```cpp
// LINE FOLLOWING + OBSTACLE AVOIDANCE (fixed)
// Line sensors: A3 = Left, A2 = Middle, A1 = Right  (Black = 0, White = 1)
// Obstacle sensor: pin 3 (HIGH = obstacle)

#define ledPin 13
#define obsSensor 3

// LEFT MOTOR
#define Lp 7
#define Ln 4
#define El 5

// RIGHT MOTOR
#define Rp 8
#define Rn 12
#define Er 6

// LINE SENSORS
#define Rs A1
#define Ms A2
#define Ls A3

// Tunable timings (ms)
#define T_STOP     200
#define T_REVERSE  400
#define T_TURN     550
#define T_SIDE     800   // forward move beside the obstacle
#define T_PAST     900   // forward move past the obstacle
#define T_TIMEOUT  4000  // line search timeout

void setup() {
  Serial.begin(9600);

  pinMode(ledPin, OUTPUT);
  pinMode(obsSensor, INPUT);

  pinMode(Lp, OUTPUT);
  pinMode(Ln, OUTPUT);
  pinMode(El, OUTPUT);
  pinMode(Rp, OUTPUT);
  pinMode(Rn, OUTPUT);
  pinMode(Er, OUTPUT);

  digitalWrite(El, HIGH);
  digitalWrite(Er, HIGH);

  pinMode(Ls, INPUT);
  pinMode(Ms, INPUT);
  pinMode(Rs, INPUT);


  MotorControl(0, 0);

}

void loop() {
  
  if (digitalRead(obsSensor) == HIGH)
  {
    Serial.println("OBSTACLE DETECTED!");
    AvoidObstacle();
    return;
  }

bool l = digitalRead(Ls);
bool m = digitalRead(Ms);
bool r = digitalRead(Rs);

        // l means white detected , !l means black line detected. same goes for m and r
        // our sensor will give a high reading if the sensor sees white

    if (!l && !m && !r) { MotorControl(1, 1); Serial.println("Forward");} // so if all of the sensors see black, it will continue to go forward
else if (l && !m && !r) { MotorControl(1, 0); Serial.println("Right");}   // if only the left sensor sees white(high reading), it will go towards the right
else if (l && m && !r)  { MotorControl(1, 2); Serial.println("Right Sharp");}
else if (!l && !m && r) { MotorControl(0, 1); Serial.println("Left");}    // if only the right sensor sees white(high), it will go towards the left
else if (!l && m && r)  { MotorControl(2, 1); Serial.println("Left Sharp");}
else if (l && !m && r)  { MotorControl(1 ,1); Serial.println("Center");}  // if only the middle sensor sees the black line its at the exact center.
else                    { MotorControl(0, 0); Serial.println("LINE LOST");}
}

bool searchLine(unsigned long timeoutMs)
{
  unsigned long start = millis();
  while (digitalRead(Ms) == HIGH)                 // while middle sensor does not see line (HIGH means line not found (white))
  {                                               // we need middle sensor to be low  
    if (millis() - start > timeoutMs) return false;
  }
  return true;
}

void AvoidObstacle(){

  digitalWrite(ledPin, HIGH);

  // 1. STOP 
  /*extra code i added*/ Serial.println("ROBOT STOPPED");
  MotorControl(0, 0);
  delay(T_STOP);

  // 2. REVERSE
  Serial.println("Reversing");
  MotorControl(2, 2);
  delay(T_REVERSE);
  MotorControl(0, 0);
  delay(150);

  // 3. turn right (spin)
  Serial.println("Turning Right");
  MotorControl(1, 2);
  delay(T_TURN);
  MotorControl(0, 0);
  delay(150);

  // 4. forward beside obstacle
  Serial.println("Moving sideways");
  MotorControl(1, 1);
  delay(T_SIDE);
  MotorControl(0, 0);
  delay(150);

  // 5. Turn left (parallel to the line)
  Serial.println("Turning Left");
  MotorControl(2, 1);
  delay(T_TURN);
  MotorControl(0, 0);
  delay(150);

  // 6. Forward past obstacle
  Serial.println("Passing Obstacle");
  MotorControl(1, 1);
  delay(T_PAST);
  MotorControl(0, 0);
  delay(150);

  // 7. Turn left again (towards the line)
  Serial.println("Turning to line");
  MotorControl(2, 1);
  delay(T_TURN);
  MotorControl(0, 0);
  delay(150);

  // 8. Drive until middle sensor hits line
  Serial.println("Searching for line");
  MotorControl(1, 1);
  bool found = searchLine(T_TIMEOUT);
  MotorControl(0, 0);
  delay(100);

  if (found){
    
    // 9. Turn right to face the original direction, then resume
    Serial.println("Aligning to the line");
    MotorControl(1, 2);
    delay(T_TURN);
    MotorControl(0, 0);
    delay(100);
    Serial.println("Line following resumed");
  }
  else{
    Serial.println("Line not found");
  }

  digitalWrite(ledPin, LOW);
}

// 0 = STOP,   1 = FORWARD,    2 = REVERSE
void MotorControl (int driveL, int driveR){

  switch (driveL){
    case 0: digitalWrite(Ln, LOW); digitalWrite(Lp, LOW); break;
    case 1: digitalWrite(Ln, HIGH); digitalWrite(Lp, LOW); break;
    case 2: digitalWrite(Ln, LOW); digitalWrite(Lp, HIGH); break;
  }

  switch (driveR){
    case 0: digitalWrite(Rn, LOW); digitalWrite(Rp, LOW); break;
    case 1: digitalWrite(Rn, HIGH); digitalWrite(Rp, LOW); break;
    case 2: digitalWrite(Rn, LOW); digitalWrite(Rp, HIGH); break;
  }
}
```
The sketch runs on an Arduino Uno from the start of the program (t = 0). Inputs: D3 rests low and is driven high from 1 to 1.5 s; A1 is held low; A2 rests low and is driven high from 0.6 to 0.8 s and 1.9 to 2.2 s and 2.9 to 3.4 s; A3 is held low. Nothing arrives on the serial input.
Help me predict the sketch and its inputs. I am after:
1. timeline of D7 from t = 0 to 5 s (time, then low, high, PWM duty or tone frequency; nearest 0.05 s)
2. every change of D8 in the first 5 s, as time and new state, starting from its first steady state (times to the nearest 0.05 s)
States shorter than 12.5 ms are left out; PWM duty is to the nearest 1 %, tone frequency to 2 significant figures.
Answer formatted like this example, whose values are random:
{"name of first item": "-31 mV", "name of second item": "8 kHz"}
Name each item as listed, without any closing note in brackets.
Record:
{"timeline of D7 from t = 0 to 5 s": "0 s low; 1.25 s high; 1.65 s low; 3.45 s high; 4 s low", "every change of D8 in the first 5 s, as time and new state, starting from its first steady state": "0 s low; 1.25 s high; 1.65 s low; 1.8 s high; 2.35 s low"}
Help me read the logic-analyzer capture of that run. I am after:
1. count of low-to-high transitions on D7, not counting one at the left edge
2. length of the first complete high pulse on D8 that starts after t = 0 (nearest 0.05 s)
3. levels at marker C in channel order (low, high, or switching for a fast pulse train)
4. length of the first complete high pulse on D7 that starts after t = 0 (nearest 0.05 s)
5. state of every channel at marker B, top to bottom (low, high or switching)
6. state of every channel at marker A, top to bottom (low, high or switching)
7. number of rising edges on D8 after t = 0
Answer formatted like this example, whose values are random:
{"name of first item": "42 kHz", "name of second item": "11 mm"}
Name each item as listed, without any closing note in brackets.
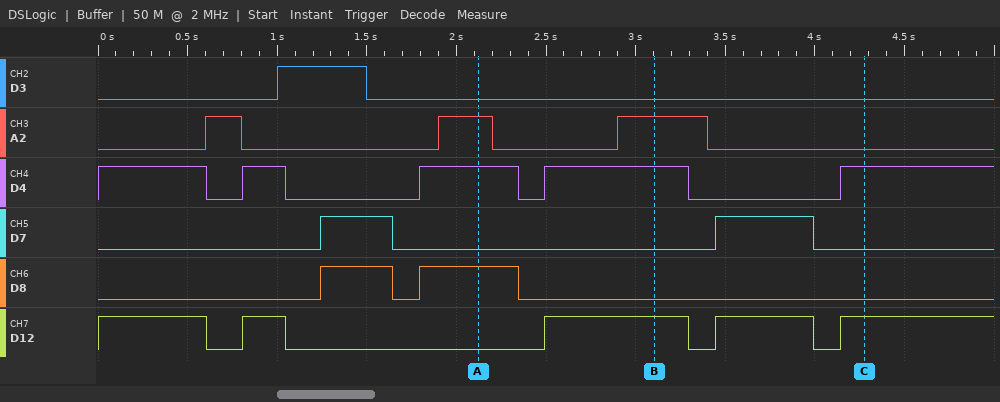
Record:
{"count of low-to-high transitions on D7, not counting one at the left edge": "2", "length of the first complete high pulse on D8 that starts after t = 0": "0.40 s", "levels at marker C in channel order": "D3 low, A2 low, D4 high, D7 low, D8 low, D12 high", "length of the first complete high pulse on D7 that starts after t = 0": "0.40 s", "state of every channel at marker B, top to bottom": "D3 low, A2 high, D4 high, D7 low, D8 low, D12 high", "state of every channel at marker A, top to bottom": "D3 low, A2 high, D4 high, D7 low, D8 high, D12 low", "number of rising edges on D8 after t = 0": "2"}
